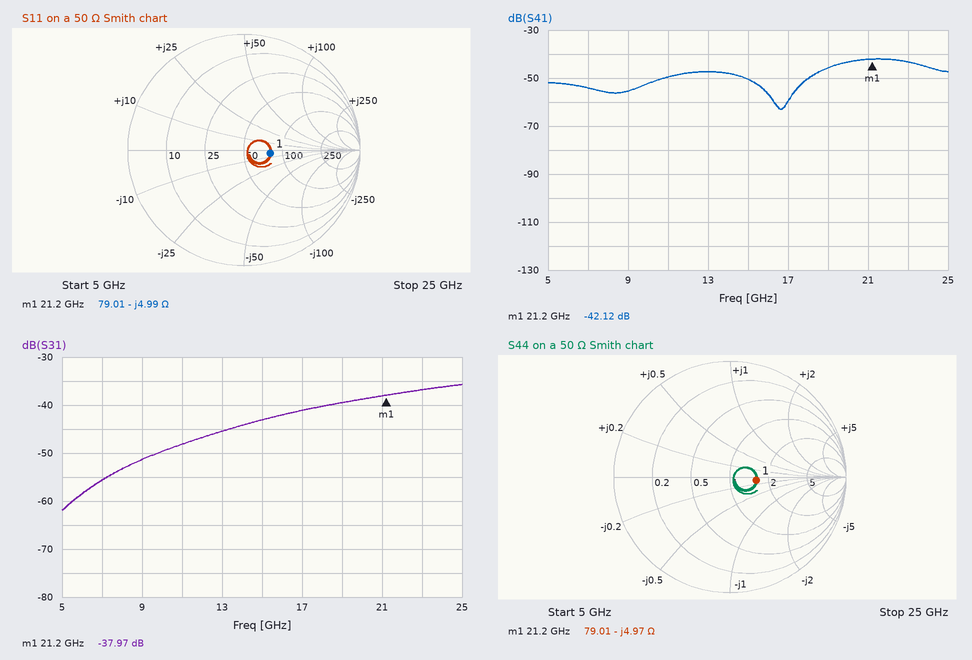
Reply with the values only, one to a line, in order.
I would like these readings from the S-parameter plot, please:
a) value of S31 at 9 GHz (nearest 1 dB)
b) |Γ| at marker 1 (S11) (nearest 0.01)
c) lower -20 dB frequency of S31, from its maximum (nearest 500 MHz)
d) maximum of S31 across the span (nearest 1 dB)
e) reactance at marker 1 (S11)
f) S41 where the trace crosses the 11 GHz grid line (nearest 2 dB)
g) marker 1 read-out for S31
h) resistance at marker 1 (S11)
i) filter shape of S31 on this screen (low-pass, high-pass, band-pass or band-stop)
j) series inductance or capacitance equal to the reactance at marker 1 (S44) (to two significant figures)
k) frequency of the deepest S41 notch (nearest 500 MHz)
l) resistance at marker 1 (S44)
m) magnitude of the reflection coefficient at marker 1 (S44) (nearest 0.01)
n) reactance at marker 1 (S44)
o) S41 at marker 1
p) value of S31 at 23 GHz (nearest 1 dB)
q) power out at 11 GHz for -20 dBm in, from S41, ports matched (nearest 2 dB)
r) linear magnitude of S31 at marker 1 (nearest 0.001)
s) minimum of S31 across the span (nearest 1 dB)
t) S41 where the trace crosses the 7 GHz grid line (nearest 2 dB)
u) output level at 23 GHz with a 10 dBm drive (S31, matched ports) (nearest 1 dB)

-51 dB
0.23
7.0 GHz
-36 dB
-4.99 Ω
-50 dB
-37.97 dB
79.01 Ω
high-pass
1.5 pF
16.5 GHz
79.01 Ω
0.23
-4.97 Ω
-42.12 dB
-37 dB
-70 dBm
0.013
-62 dB
-54 dB
-27 dBm
